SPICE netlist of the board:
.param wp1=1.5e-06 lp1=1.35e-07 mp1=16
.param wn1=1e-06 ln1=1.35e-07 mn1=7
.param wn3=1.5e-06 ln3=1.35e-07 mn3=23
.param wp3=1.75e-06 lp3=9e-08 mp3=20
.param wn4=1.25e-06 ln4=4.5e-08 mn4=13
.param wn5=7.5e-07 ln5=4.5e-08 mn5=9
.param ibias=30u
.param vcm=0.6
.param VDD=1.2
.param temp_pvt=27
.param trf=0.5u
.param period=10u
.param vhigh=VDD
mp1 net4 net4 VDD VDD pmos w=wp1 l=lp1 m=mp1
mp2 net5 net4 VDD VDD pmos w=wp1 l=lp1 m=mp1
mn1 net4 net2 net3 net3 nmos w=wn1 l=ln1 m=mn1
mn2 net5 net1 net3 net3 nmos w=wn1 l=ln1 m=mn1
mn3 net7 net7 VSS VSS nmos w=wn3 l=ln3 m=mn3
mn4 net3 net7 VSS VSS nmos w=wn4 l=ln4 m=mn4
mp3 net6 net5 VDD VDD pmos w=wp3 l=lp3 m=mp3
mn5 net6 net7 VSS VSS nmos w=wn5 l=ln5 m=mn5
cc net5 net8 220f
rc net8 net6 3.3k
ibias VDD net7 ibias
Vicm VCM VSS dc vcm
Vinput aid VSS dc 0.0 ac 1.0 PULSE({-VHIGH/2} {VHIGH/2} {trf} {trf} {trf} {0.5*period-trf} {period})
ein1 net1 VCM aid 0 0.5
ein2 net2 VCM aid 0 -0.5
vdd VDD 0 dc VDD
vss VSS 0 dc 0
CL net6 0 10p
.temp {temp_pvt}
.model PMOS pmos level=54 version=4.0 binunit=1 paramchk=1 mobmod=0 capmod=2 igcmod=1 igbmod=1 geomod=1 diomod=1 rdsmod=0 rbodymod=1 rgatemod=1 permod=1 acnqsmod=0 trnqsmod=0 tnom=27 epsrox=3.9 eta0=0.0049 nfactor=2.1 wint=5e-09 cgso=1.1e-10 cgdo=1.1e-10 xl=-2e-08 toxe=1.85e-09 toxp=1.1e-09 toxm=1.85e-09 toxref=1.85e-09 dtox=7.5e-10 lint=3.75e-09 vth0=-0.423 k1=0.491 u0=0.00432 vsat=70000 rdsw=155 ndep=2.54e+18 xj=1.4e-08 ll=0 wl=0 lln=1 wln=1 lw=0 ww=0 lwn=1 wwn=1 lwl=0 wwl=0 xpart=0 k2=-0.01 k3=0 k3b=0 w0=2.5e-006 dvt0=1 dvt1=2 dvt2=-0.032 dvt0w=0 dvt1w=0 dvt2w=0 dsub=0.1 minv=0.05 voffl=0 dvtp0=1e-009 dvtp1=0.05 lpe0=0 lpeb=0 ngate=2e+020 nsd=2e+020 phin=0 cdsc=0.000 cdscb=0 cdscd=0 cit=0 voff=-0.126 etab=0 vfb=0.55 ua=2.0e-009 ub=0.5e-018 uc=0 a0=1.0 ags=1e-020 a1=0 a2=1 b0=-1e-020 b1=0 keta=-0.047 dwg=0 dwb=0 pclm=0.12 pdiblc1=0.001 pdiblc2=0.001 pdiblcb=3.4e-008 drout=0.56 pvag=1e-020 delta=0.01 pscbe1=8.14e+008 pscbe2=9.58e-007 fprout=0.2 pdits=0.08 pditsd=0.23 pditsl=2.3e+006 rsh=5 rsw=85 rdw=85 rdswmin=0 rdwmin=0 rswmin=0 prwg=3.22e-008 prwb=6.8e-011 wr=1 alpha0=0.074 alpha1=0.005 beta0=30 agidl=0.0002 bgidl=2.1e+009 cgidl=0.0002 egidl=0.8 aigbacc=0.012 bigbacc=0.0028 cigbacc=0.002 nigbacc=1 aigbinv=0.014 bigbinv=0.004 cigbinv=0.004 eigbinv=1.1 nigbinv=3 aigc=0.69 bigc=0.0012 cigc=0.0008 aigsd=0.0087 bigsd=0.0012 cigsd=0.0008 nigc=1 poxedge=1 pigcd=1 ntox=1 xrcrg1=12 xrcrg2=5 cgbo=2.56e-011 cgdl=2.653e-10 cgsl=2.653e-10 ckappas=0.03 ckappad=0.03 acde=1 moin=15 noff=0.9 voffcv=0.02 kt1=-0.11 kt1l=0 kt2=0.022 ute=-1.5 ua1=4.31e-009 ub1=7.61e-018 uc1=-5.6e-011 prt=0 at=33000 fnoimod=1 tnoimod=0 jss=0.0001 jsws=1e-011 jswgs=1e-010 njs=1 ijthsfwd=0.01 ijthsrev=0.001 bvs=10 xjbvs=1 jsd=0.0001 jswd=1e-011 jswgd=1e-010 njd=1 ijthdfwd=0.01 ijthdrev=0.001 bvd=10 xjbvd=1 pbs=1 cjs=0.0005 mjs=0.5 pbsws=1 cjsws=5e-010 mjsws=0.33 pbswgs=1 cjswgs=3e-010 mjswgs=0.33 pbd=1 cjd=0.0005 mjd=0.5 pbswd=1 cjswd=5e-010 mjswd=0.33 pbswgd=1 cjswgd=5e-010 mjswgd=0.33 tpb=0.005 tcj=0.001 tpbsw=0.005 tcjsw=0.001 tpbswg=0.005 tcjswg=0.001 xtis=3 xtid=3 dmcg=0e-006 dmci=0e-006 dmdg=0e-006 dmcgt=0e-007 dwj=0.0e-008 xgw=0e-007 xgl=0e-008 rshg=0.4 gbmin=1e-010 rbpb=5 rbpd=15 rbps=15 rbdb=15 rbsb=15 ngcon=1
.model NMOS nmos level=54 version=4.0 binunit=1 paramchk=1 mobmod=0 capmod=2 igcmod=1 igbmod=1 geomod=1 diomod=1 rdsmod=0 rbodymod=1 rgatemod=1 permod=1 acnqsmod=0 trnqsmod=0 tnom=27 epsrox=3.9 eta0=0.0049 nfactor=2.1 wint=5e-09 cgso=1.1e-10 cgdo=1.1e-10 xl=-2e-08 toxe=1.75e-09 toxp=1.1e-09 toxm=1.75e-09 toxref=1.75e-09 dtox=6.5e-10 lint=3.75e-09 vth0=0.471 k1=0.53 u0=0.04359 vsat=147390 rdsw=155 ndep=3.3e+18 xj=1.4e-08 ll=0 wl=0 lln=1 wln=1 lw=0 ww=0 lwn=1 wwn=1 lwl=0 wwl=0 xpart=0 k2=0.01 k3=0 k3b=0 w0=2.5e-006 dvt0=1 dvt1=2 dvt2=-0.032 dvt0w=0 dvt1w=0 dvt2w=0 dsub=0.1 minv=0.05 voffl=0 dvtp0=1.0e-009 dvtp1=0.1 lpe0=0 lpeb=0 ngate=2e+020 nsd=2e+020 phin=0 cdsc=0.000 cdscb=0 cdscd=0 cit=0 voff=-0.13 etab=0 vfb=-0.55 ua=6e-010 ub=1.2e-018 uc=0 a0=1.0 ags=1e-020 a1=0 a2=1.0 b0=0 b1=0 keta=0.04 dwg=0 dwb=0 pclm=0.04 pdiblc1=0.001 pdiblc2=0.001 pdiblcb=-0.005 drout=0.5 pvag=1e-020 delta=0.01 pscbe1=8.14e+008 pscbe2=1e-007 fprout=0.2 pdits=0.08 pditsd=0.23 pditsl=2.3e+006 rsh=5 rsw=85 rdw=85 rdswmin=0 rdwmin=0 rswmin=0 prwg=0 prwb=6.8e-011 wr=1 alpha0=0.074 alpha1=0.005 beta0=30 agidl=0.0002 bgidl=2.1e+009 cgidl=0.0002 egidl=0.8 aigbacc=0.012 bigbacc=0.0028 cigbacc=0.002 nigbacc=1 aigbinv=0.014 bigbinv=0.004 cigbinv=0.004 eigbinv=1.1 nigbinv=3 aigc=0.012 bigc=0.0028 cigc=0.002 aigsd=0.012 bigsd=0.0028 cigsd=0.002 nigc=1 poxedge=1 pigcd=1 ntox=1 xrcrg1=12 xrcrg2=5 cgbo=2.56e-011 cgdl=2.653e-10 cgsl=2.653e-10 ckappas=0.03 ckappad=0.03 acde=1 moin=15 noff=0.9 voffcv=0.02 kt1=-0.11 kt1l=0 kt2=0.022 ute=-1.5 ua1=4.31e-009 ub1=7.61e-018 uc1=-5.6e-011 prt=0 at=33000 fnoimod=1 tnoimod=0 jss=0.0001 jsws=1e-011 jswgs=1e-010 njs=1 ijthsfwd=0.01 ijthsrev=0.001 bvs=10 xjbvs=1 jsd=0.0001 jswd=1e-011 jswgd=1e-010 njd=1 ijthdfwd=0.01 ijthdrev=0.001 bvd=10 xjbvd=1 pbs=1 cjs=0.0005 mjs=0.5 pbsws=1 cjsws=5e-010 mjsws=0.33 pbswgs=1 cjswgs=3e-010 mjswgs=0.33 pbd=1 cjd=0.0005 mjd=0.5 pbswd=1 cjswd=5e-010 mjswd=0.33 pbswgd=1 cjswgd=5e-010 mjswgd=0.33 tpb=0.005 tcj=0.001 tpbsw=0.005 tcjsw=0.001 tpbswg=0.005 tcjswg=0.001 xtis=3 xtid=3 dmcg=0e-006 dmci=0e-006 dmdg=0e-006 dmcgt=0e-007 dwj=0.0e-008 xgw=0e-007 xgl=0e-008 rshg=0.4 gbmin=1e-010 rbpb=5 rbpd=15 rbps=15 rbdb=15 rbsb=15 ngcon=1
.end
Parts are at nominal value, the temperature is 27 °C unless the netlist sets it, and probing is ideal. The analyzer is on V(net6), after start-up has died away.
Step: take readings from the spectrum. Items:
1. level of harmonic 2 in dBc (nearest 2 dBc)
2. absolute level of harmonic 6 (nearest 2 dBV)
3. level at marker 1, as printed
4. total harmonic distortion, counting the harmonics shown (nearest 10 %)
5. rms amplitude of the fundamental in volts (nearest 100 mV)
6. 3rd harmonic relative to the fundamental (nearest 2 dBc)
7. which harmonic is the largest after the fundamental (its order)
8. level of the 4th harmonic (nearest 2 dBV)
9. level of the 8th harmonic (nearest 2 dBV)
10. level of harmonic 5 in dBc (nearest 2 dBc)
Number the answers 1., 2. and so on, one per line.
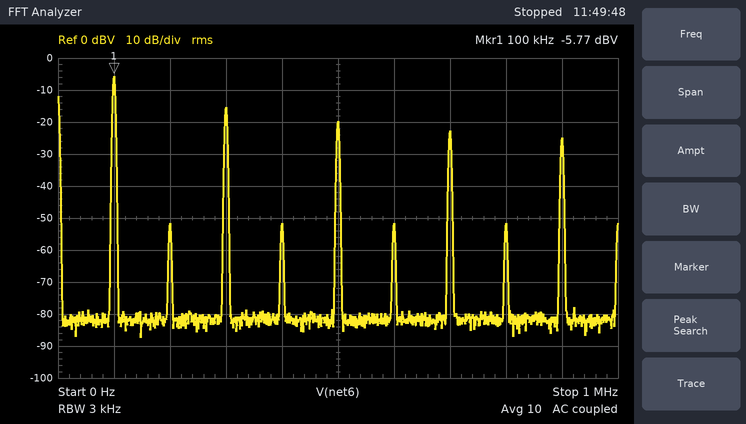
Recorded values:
1. -46 dBc
2. -52 dBV
3. -5.77 dBV
4. 40 %
5. 500 mV
6. -10 dBc
7. 3
8. -52 dBV
9. -52 dBV
10. -14 dBc
